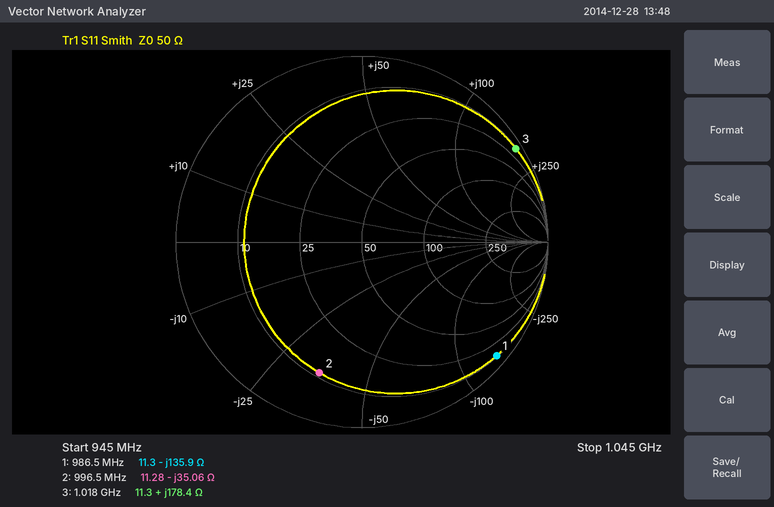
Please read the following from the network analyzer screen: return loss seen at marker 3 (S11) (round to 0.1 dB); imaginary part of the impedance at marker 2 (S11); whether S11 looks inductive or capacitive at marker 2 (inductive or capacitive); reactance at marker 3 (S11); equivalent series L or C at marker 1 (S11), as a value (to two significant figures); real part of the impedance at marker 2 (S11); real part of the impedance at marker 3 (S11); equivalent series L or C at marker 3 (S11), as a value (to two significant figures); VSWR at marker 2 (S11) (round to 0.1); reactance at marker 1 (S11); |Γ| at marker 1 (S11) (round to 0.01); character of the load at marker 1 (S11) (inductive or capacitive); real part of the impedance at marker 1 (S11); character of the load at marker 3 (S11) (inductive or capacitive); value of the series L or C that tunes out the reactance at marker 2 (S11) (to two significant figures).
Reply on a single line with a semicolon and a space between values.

0.3 dB; -35.06 Ω; capacitive; +178.4 Ω; 1.2 pF; 11.28 Ω; 11.3 Ω; 28 nH; 6.7; -135.9 Ω; 0.95; capacitive; 11.3 Ω; inductive; 5.6 nH
